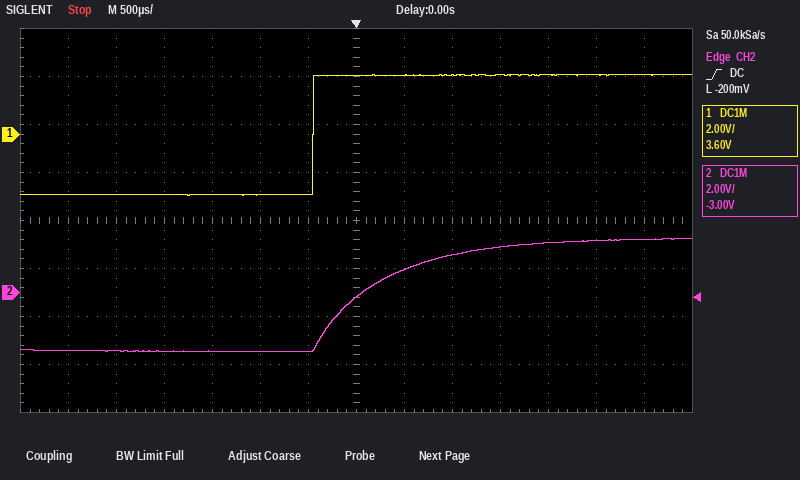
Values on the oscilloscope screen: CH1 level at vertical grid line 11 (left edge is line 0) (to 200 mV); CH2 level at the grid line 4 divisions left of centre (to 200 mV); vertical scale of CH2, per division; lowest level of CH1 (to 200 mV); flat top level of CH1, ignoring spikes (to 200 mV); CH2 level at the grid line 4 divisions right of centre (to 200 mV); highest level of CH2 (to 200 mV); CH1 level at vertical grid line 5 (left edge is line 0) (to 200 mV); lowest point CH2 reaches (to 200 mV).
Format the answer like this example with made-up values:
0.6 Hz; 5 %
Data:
2.4 V; -2.4 V; 2 V; -2.6 V; 2.4 V; 2.0 V; 2.2 V; -2.6 V; -2.4 V
